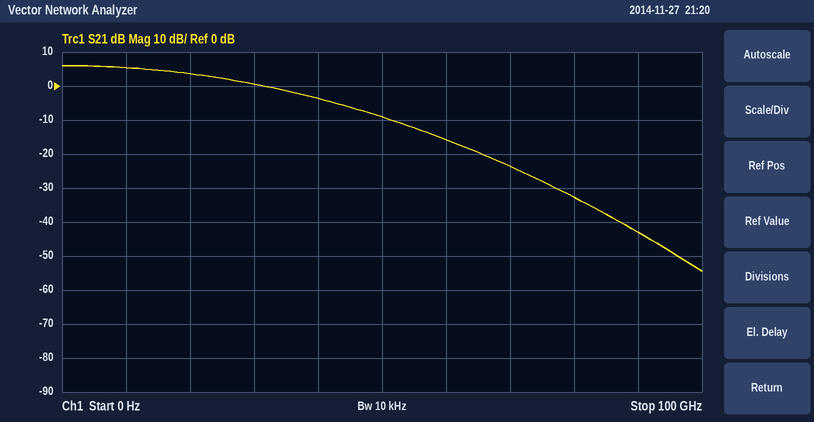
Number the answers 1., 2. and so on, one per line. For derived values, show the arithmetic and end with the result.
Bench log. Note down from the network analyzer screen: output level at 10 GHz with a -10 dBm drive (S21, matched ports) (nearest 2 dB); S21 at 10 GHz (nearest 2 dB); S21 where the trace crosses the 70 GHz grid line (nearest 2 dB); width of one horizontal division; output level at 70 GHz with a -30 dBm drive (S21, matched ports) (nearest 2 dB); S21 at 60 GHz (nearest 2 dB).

1. -10 dBm + (6 dB) = -4 dBm
2. 6 dB
3. -24 dB
4. 10 GHz
5. -30 dBm + (-24 dB) = -54 dBm
6. -16 dB
